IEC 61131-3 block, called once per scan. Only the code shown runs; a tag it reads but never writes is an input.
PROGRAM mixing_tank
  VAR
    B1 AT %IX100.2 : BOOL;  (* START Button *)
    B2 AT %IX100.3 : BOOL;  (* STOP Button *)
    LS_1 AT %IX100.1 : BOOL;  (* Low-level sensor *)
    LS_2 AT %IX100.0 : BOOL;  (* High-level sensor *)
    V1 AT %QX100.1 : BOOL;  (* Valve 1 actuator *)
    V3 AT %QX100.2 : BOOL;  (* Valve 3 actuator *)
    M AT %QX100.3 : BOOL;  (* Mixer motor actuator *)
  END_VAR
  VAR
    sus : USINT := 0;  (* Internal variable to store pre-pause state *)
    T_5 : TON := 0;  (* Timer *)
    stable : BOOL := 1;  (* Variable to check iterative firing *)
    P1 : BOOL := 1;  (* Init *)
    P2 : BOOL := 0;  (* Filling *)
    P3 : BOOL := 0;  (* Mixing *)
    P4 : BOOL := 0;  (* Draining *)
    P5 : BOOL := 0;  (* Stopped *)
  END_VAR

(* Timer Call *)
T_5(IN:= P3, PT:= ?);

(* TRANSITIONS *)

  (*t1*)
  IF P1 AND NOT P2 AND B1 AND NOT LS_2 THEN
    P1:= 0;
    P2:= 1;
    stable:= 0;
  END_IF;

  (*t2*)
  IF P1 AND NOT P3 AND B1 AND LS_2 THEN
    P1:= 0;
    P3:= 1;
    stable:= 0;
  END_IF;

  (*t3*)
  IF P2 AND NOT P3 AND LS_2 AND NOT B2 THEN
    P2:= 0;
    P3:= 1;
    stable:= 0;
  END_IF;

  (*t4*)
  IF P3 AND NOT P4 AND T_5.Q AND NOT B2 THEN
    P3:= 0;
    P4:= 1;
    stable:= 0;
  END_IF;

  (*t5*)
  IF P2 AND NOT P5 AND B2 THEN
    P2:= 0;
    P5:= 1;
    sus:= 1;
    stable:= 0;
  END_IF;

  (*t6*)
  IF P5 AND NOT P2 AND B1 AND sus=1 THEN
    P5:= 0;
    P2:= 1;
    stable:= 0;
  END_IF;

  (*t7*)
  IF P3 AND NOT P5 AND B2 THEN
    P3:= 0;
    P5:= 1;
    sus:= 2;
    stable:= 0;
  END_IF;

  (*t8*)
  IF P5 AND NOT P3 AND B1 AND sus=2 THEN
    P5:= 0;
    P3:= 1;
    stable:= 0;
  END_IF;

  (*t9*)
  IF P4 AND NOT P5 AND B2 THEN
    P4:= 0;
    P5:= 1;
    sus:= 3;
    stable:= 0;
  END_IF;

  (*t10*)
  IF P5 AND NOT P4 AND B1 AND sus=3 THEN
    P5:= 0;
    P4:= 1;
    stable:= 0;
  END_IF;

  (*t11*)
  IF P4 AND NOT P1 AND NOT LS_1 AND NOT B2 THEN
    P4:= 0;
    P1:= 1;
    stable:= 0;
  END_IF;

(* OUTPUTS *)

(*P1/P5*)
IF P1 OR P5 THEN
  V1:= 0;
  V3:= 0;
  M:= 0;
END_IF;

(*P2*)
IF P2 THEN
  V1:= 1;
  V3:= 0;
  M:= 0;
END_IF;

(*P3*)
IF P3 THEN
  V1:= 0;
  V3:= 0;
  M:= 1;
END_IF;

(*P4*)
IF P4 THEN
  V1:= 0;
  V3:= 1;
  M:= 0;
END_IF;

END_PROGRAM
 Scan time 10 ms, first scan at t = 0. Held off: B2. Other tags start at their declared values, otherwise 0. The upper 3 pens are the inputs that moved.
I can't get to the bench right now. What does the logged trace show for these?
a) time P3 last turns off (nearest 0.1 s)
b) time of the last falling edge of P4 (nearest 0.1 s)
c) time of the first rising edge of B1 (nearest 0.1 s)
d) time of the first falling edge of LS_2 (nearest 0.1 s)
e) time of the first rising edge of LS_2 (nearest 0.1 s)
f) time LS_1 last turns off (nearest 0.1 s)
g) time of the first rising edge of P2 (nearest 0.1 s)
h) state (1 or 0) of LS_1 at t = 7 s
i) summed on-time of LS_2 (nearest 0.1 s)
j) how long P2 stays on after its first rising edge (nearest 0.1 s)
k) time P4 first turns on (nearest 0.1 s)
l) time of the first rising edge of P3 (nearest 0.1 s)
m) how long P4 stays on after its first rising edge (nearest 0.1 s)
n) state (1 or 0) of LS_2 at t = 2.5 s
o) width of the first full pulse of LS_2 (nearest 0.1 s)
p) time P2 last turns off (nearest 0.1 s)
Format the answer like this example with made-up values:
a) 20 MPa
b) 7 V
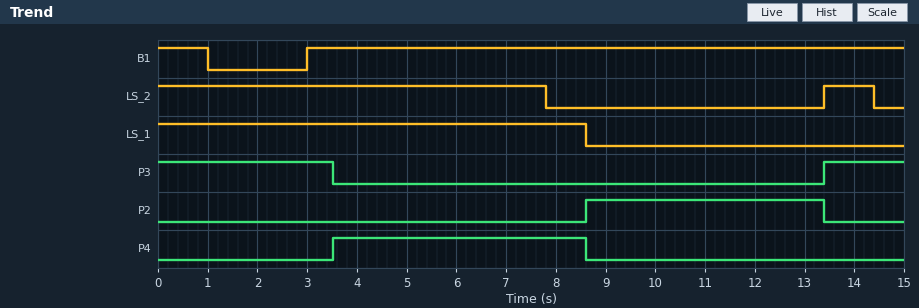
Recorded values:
a) 3.5 s
b) 8.6 s
c) 3.0 s
d) 7.8 s
e) 13.4 s
f) 8.6 s
g) 8.6 s
h) 1
i) 8.8 s
j) 4.8 s
k) 3.5 s
l) 13.4 s
m) 5.1 s
n) 1
o) 1.0 s
p) 13.4 s
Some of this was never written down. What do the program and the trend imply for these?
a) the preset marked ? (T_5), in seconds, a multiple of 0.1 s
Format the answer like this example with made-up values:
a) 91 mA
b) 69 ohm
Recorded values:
a) 3.5 s
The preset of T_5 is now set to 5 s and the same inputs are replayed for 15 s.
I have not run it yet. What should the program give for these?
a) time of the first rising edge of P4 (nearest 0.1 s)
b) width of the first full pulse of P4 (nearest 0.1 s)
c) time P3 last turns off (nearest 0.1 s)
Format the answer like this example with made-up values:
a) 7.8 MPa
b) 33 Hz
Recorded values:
a) 5.0 s
b) 3.6 s
c) 5.0 s
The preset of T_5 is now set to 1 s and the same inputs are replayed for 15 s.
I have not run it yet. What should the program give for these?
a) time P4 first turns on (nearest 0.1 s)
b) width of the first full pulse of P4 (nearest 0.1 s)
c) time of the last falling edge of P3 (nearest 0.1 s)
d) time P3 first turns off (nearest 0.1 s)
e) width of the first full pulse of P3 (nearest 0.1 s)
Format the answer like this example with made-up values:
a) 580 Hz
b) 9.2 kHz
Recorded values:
a) 1.0 s
b) 7.6 s
c) 14.4 s
d) 1.0 s
e) 1.0 s
